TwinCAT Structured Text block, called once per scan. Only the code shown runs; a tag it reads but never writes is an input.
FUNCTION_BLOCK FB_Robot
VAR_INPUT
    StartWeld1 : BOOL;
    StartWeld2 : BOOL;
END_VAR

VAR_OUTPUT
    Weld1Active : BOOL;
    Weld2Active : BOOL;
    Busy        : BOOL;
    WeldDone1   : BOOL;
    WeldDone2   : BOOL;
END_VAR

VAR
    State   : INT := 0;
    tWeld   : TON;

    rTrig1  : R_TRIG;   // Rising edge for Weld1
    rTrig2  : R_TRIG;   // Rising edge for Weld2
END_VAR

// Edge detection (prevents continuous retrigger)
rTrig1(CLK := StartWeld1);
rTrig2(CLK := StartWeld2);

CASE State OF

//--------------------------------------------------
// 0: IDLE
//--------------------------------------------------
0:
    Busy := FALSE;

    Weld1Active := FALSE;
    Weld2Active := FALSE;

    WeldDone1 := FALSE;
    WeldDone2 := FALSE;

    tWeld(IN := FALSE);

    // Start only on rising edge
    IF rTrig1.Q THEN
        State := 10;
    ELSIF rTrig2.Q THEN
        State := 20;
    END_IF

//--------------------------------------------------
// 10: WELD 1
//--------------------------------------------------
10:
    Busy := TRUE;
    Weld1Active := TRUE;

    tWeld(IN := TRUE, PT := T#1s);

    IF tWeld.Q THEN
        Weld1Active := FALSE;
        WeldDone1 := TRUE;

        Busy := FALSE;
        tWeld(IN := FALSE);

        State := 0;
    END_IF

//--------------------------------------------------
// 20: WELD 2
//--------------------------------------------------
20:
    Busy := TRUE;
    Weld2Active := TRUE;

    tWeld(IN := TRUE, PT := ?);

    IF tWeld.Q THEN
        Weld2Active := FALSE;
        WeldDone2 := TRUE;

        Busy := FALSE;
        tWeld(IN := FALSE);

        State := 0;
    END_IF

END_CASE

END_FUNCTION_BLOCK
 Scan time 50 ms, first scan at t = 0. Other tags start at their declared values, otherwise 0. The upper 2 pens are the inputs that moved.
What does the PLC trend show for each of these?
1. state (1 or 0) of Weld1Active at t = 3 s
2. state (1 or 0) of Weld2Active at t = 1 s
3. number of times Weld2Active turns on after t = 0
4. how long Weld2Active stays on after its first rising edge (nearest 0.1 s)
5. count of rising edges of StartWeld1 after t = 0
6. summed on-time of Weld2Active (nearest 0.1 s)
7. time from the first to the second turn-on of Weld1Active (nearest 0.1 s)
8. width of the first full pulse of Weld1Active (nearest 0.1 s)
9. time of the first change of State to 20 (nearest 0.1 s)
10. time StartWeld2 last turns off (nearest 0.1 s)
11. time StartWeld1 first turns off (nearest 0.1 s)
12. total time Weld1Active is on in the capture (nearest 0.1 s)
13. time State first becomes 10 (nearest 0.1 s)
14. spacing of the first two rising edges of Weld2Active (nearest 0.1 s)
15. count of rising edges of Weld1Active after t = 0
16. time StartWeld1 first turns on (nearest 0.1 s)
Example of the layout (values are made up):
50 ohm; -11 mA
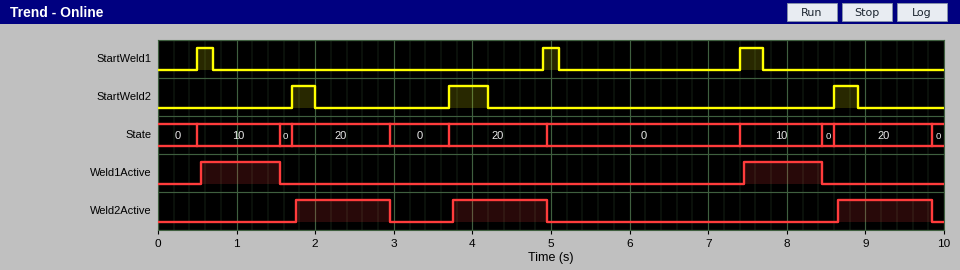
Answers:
0; 0; 3; 1.2 s; 3; 3.6 s; 6.9 s; 1.0 s; 1.7 s; 8.9 s; 0.7 s; 2.0 s; 0.5 s; 2.0 s; 2; 0.5 s
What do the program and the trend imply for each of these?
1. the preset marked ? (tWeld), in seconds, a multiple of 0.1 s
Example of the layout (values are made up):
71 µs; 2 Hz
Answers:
1.2 s
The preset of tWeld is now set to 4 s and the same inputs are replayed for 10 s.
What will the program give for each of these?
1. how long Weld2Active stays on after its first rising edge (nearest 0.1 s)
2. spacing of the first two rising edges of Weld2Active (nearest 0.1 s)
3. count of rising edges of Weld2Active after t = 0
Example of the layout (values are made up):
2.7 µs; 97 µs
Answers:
4.0 s; 6.9 s; 2
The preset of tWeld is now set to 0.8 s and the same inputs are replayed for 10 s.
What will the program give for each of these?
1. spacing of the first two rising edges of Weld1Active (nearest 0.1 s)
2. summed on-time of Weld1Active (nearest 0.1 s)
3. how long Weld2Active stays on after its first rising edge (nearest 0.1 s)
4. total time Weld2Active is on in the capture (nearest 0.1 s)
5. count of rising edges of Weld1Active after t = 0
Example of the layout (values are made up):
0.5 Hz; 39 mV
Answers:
4.4 s; 3.0 s; 0.8 s; 2.4 s; 3
